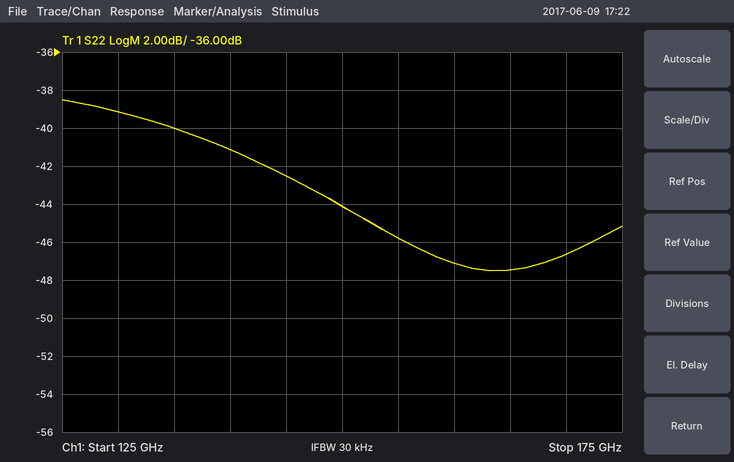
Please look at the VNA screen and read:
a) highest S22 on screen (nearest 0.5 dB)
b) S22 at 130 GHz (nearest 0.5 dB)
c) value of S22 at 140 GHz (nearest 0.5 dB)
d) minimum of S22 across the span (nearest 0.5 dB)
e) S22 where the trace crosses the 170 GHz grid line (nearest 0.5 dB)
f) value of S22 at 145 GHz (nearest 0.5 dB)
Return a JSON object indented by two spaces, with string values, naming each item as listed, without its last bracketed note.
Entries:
{
  "highest S22 on screen": "-38.5 dB",
  "S22 at 130 GHz": "-39.0 dB",
  "value of S22 at 140 GHz": "-41.0 dB",
  "minimum of S22 across the span": "-47.5 dB",
  "S22 where the trace crosses the 170 GHz grid line": "-46.5 dB",
  "value of S22 at 145 GHz": "-42.5 dB"
}
